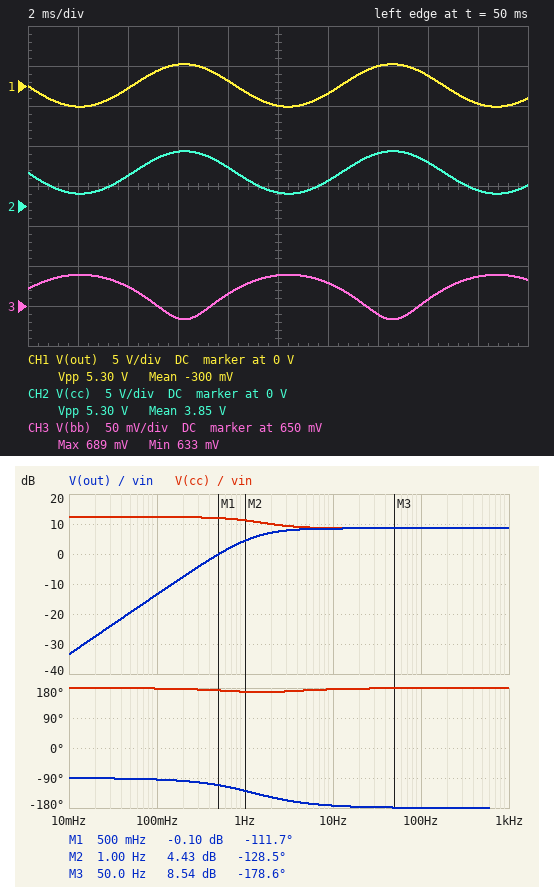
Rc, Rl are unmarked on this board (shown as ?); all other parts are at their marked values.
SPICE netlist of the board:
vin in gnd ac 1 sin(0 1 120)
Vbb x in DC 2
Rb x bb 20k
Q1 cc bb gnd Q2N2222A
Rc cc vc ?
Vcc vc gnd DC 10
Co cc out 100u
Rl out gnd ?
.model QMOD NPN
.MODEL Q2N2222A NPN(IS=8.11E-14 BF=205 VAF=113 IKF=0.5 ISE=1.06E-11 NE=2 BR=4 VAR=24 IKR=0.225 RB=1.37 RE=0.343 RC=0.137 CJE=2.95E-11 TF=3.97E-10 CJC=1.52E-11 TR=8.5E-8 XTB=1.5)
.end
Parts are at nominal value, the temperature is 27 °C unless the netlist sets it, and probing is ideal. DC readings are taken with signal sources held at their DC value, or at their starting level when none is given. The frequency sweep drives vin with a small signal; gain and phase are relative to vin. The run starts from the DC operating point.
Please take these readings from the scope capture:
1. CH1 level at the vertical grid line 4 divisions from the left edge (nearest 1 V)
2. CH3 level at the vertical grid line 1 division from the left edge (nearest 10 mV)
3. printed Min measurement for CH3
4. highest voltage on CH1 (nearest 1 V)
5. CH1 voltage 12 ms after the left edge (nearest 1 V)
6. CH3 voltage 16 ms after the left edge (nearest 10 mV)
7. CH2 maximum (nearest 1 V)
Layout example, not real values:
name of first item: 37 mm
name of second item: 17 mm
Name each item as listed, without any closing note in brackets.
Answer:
CH1 level at the vertical grid line 4 divisions from the left edge: 1 V
CH3 level at the vertical grid line 1 division from the left edge: 690 mV
printed Min measurement for CH3: 633 mV
highest voltage on CH1: 3 V
CH1 voltage 12 ms after the left edge: -1 V
CH3 voltage 16 ms after the left edge: 660 mV
CH2 maximum: 7 V
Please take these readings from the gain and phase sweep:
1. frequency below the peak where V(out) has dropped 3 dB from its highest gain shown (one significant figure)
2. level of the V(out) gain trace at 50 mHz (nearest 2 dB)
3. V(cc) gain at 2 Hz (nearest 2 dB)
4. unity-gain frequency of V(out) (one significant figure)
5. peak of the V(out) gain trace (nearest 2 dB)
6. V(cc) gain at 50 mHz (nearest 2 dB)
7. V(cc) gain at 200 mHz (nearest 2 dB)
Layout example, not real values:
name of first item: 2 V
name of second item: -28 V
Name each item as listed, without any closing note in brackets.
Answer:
frequency below the peak where V(out) has dropped 3 dB from its highest gain shown: 1 Hz
level of the V(out) gain trace at 50 mHz: -20 dB
V(cc) gain at 2 Hz: 10 dB
unity-gain frequency of V(out): 500 mHz
peak of the V(out) gain trace: 8 dB
V(cc) gain at 50 mHz: 12 dB
V(cc) gain at 200 mHz: 12 dB
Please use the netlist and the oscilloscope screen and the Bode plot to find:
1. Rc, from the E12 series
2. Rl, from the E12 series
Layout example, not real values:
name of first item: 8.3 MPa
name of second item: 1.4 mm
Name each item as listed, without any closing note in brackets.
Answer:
Rc, from the E12 series: 470 Ω
Rl, from the E12 series: 820 Ω
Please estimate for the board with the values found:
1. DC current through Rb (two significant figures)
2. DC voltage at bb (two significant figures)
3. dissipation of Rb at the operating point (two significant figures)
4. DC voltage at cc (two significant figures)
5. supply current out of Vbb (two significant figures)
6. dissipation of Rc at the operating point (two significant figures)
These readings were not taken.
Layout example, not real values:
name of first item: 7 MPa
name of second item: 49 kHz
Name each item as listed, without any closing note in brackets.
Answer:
DC current through Rb: 66 µA
DC voltage at bb: 670 mV
dissipation of Rb at the operating point: 88 µW
DC voltage at cc: 4.1 V
supply current out of Vbb: 66 µA
dissipation of Rc at the operating point: 73 mW
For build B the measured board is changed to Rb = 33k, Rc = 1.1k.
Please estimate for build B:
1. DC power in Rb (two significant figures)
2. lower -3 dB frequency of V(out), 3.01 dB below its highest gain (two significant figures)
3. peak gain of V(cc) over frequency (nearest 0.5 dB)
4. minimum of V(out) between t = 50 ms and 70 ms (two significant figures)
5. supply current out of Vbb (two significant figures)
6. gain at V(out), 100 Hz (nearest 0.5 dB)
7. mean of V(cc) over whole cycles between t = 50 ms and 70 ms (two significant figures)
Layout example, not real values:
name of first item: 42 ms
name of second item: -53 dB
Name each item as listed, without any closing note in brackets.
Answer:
DC power in Rb: 55 µW
lower -3 dB frequency of V(out), 3.01 dB below its highest gain: 860 mHz
peak gain of V(cc) over frequency: 15.0 dB
minimum of V(out) between t = 50 ms and 70 ms: -1.8 V
supply current out of Vbb: 41 µA
gain at V(out), 100 Hz: 8.0 dB
mean of V(cc) over whole cycles between t = 50 ms and 70 ms: 2.0 V
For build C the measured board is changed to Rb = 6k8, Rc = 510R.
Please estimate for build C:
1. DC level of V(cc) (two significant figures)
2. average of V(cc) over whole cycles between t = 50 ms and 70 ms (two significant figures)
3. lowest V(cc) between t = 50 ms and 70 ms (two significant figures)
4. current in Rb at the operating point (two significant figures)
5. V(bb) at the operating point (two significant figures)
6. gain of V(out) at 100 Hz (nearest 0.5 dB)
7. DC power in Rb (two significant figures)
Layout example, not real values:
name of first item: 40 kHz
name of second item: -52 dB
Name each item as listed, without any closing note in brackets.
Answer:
DC level of V(cc): 120 mV
average of V(cc) over whole cycles between t = 50 ms and 70 ms: 780 mV
lowest V(cc) between t = 50 ms and 70 ms: 93 mV
current in Rb at the operating point: 190 µA
V(bb) at the operating point: 690 mV
gain of V(out) at 100 Hz: -27.5 dB
DC power in Rb: 250 µW
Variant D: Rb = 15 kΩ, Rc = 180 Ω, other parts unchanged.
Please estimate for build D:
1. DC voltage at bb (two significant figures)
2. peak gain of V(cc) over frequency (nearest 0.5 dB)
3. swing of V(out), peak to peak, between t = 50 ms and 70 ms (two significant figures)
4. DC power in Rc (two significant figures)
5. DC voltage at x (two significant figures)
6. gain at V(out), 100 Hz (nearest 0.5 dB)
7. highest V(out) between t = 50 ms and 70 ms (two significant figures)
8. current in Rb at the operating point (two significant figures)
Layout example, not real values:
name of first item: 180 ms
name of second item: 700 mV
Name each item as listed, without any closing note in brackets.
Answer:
DC voltage at bb: 680 mV
peak gain of V(cc) over frequency: 7.0 dB
swing of V(out), peak to peak, between t = 50 ms and 70 ms: 3.6 V
DC power in Rc: 52 mW
DC voltage at x: 2.0 V
gain at V(out), 100 Hz: 5.0 dB
highest V(out) between t = 50 ms and 70 ms: 1.8 V
current in Rb at the operating point: 88 µA
